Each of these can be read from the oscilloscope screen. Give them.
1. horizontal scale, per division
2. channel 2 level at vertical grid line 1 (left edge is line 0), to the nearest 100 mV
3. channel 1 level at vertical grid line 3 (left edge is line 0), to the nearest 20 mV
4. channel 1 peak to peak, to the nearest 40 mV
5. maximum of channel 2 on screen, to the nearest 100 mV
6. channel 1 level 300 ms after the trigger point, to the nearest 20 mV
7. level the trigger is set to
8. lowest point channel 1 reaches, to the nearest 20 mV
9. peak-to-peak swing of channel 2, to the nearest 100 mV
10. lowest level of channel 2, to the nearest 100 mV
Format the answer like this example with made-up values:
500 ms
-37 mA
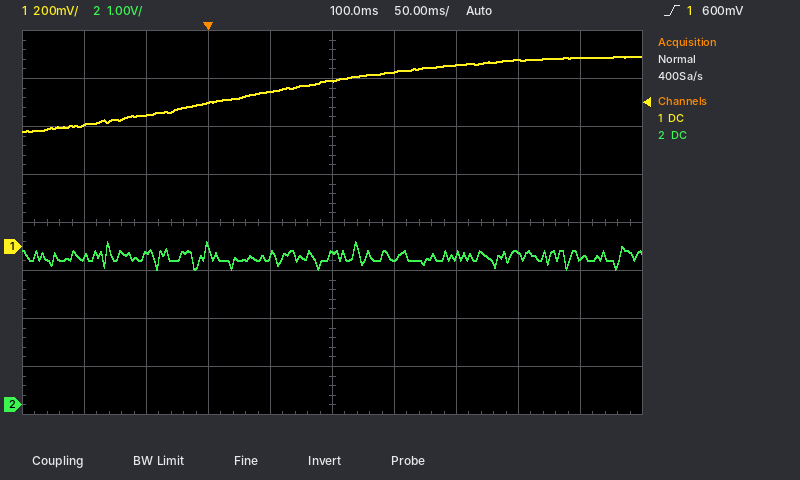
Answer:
50 ms
3.1 V
600 mV
320 mV
3.4 V
780 mV
600 mV
480 mV
600 mV
2.8 V
